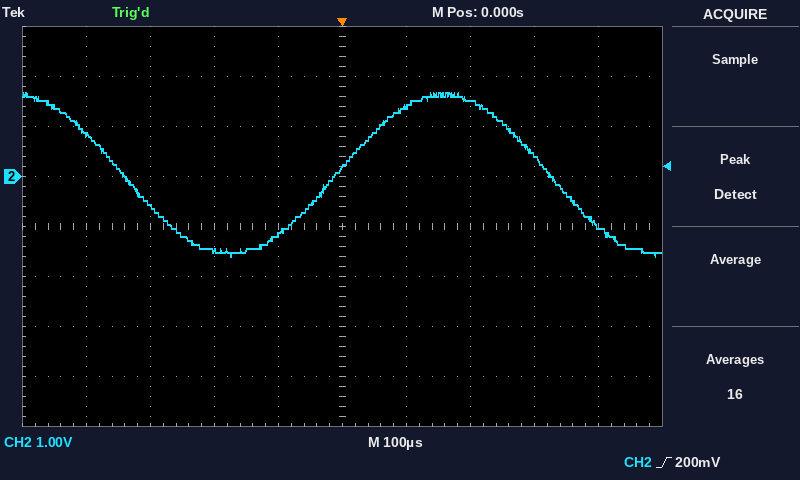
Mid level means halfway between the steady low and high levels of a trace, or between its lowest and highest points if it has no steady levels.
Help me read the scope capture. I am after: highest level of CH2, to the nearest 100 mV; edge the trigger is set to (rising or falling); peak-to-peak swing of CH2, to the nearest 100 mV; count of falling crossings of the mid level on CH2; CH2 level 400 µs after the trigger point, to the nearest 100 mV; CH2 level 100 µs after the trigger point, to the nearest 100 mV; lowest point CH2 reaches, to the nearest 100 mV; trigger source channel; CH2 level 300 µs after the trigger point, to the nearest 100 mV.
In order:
1.7 V
rising
3.3 V
2
-1.0 V
1.4 V
-1.6 V
CH2
400 mV
